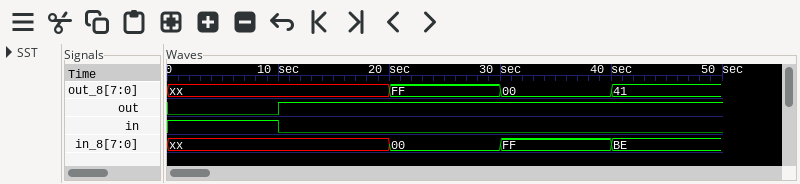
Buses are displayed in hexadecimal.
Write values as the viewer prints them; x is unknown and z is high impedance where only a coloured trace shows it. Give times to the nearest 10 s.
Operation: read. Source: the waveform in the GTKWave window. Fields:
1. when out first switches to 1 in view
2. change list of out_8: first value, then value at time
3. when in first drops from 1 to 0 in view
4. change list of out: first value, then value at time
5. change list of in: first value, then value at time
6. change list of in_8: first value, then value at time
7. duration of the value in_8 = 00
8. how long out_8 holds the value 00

10 s
xx, FF at 20 s, 00 at 30 s, 41 at 40 s
10 s
0, 1 at 10 s
1, 0 at 10 s
xx, 00 at 20 s, FF at 30 s, BE at 40 s
10 s
10 s
